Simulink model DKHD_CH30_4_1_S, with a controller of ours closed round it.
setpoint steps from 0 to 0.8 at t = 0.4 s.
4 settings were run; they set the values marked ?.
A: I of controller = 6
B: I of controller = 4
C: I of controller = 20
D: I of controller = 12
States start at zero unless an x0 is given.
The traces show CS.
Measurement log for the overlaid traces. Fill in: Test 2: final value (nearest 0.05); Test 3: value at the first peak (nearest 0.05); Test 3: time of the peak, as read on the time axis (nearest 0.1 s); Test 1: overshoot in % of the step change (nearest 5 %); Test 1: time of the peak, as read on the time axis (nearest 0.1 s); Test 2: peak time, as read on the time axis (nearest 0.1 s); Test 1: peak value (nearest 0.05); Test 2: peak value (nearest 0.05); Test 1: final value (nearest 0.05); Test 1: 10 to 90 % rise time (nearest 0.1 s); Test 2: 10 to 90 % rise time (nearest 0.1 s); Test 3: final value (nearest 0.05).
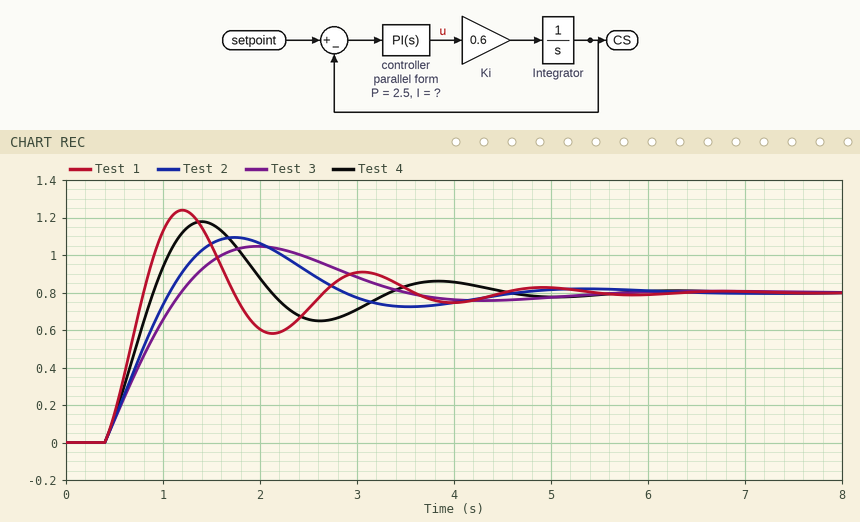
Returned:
0.80
1.05
2.0 s
55 %
1.2 s
1.7 s
1.25
1.10
0.80
0.3 s
0.5 s
0.80
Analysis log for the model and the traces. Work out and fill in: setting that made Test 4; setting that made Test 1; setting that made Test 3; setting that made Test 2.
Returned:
D
C
B
A
